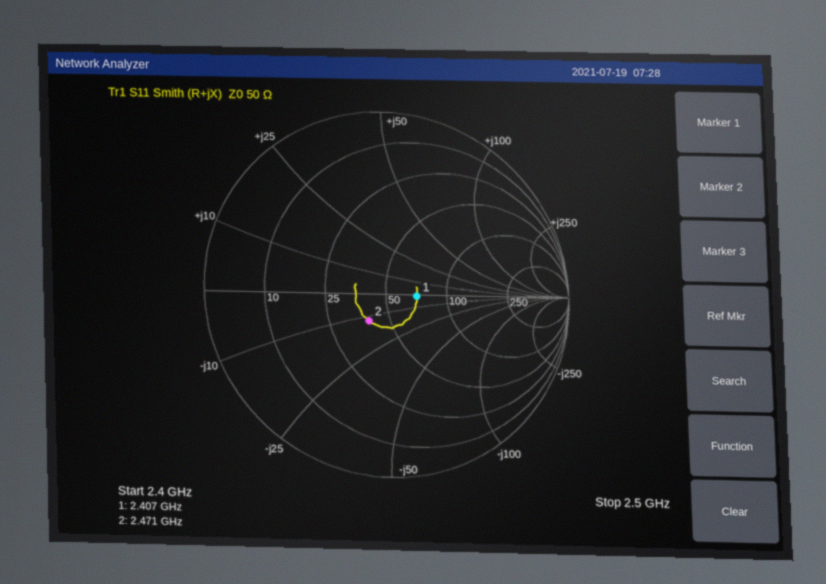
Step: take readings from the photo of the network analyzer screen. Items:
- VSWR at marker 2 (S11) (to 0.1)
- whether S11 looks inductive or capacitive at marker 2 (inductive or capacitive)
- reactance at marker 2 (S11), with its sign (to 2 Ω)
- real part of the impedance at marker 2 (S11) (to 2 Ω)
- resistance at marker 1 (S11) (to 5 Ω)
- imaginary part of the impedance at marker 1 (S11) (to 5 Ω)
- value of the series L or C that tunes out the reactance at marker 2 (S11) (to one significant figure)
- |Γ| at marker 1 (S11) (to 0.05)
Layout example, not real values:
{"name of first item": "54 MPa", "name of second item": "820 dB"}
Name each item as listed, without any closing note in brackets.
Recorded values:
{"VSWR at marker 2 (S11)": "1.4", "whether S11 looks inductive or capacitive at marker 2": "capacitive", "reactance at marker 2 (S11), with its sign": "-12 Ω", "real part of the impedance at marker 2 (S11)": "40 Ω", "resistance at marker 1 (S11)": "70 Ω", "imaginary part of the impedance at marker 1 (S11)": "0 Ω", "value of the series L or C that tunes out the reactance at marker 2 (S11)": "800 pH", "|Γ| at marker 1 (S11)": "0.15"}
